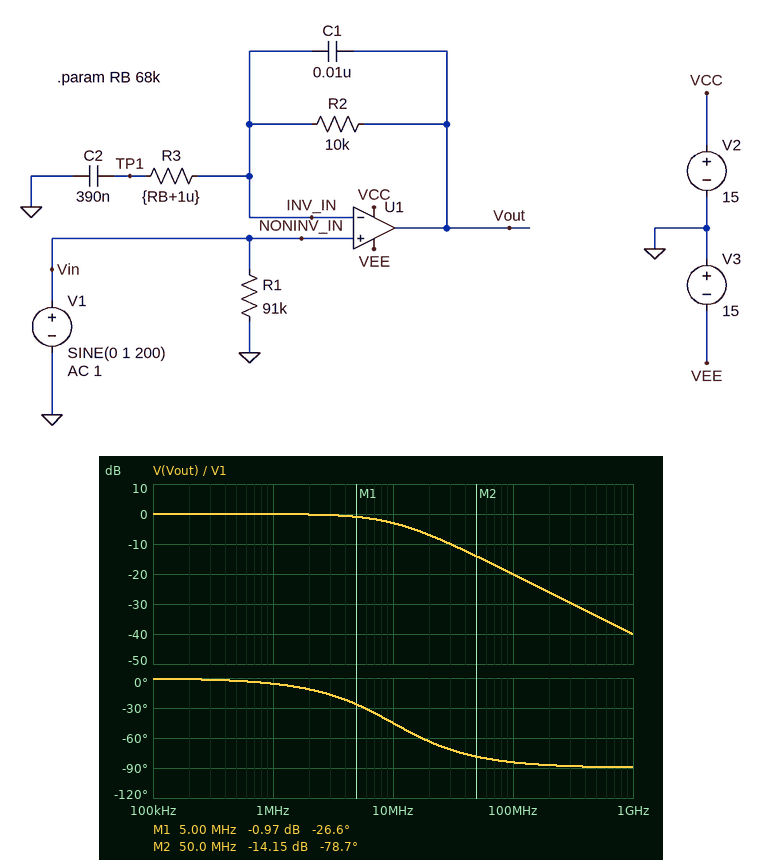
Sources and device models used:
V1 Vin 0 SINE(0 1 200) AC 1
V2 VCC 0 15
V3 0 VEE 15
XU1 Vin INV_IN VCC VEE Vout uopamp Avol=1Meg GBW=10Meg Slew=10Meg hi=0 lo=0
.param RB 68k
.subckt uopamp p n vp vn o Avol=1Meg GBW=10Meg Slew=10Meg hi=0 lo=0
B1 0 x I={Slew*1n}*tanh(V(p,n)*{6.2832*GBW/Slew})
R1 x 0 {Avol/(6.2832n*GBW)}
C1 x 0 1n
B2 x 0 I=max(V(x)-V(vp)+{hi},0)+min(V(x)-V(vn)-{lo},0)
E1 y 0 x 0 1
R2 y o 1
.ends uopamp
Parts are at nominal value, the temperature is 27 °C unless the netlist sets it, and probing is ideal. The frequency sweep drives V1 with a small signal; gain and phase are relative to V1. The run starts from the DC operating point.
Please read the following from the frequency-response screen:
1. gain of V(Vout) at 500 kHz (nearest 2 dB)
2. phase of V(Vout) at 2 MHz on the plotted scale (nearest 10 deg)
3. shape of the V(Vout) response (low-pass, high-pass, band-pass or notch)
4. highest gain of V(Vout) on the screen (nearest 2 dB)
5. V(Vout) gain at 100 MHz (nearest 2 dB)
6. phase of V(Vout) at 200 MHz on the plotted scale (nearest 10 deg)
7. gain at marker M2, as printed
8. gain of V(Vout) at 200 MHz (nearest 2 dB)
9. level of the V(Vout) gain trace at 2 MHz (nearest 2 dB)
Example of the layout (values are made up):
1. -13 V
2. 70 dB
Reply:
1. 0 dB
2. -10 deg
3. low-pass
4. 0 dB
5. -20 dB
6. -90 deg
7. -14.15 dB
8. -26 dB
9. 0 dB
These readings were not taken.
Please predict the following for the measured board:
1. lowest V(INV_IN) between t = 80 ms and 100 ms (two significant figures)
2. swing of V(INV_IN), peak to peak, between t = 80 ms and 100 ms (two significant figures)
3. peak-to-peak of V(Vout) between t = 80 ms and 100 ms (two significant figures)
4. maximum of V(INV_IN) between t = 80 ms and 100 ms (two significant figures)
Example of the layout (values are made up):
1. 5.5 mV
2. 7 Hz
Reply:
1. -1.0 V
2. 2.0 V
3. 2.3 V
4. 1.0 V
